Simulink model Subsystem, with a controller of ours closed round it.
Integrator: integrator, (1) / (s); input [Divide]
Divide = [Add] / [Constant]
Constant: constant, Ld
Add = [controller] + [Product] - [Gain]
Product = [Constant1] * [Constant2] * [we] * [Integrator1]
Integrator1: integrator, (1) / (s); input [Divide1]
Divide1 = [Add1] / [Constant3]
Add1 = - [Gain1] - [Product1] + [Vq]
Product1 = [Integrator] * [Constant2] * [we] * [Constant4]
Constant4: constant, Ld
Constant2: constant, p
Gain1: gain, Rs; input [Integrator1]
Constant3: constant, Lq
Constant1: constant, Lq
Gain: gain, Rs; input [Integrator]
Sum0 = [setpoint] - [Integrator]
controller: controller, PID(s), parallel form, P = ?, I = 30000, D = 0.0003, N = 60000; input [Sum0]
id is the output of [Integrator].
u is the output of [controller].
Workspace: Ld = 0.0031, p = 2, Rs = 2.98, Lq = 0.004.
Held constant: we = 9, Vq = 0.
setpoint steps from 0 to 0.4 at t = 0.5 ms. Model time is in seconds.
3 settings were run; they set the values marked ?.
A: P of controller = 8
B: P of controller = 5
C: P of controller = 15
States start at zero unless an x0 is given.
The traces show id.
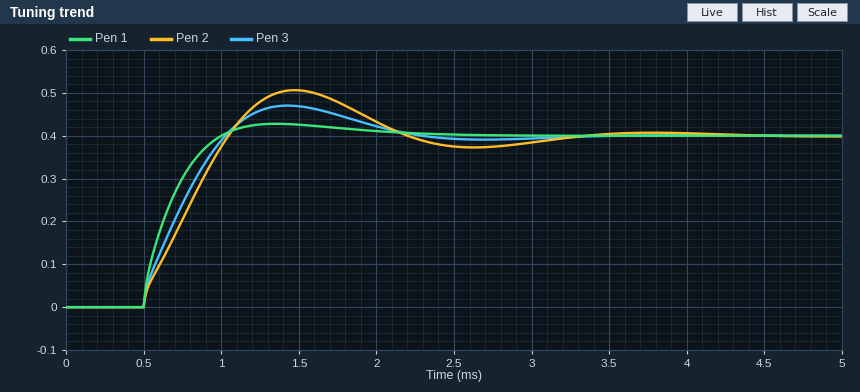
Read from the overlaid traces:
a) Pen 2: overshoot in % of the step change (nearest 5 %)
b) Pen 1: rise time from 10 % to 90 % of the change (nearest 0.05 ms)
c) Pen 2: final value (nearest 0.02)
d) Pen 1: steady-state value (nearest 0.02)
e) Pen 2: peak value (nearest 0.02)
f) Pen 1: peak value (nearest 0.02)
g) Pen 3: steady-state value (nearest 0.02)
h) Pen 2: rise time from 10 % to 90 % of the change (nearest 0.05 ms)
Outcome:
25 %
0.35 ms
0.40
0.40
0.50
0.42
0.40
0.45 ms
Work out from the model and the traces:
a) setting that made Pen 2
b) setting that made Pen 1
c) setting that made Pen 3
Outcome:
B
C
A
